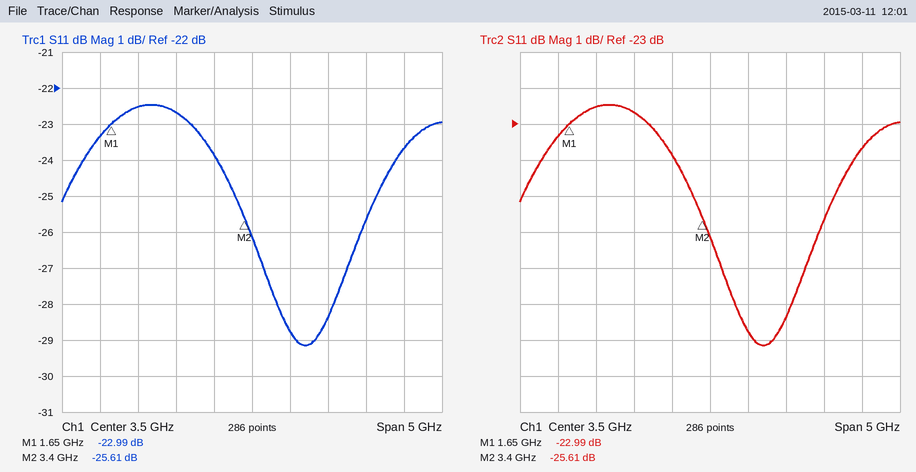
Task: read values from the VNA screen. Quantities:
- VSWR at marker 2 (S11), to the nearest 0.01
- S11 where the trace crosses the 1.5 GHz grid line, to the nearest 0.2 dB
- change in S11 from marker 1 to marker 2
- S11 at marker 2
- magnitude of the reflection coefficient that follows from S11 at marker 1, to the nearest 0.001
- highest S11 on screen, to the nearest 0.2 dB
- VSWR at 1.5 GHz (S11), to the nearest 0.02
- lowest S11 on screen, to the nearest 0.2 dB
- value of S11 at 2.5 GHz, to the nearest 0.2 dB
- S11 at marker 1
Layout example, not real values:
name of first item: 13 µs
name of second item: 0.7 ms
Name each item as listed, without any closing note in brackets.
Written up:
VSWR at marker 2 (S11), to the nearest 0.01: 1.11
S11 where the trace crosses the 1.5 GHz grid line, to the nearest 0.2 dB: -23.4 dB
change in S11 from marker 1 to marker 2: -2.62 dB
S11 at marker 2: -25.61 dB
magnitude of the reflection coefficient that follows from S11 at marker 1, to the nearest 0.001: 0.071
highest S11 on screen, to the nearest 0.2 dB: -22.4 dB
VSWR at 1.5 GHz (S11), to the nearest 0.02: 1.14
lowest S11 on screen, to the nearest 0.2 dB: -29.2 dB
value of S11 at 2.5 GHz, to the nearest 0.2 dB: -22.6 dB
S11 at marker 1: -22.99 dB
